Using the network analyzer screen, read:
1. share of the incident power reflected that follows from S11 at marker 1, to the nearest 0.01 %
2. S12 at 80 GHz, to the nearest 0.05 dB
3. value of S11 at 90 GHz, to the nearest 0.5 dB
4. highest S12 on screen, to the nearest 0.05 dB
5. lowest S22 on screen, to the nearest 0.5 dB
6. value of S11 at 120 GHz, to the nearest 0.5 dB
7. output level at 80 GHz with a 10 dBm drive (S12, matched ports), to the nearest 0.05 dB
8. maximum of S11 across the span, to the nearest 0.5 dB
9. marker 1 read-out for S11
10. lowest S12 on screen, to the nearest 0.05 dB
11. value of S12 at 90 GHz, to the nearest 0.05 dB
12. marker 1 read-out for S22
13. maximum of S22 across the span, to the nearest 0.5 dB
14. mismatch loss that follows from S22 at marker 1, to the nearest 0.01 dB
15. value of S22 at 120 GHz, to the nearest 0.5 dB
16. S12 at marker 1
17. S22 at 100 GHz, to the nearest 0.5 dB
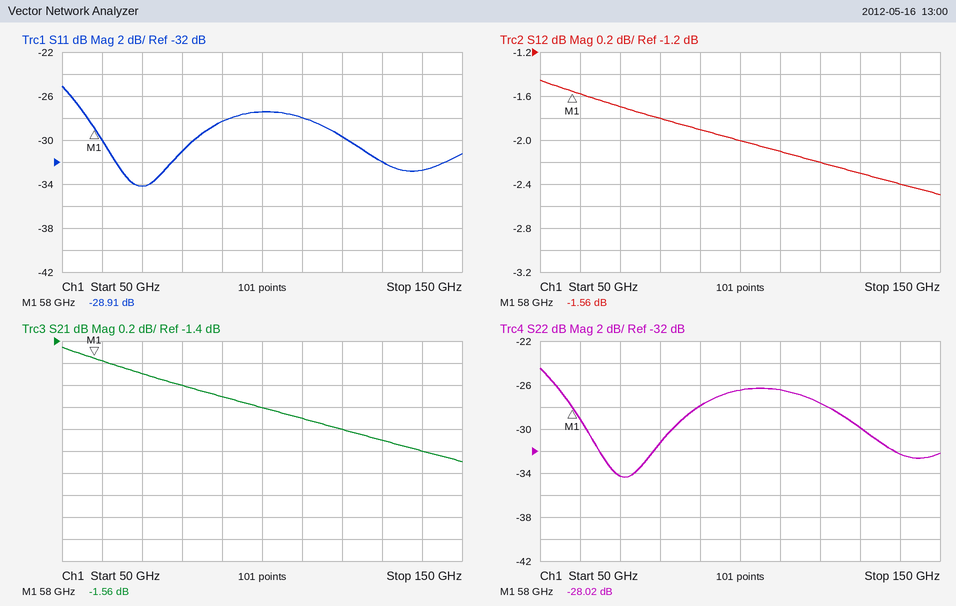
0.13 %
-1.80 dB
-28.5 dB
-1.45 dB
-34.5 dB
-29.5 dB
8.20 dBm
-25.0 dB
-28.91 dB
-2.50 dB
-1.90 dB
-28.02 dB
-24.5 dB
0.01 dB
-27.5 dB
-1.56 dB
-26.5 dB
